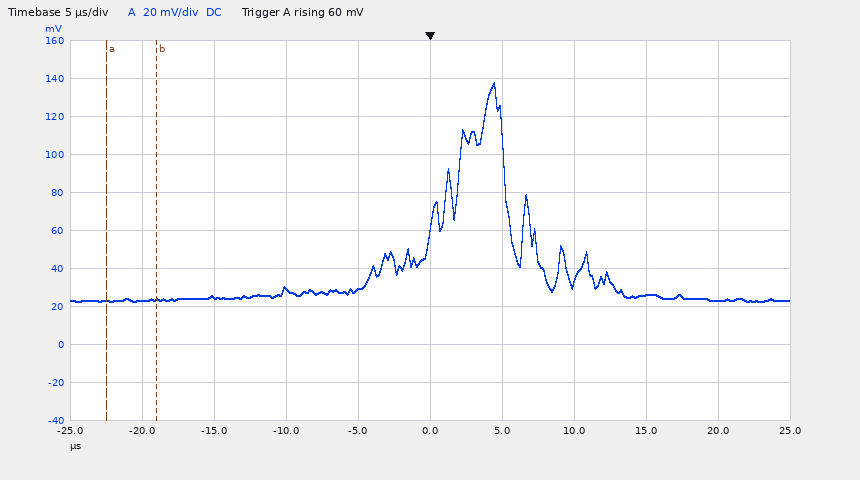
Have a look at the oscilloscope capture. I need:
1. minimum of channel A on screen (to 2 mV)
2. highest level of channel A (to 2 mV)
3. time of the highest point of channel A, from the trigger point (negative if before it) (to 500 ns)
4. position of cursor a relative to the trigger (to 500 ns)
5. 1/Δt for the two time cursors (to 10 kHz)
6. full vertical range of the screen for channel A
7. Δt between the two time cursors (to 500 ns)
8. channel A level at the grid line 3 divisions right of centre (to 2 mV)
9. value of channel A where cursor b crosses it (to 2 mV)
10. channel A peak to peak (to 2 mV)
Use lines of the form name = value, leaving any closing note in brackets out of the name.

minimum of channel A on screen = 22 mV
highest level of channel A = 138 mV
time of the highest point of channel A, from the trigger point (negative if before it) = +4.5 µs
position of cursor a relative to the trigger = -22.5 µs
1/Δt for the two time cursors = 290 kHz
full vertical range of the screen for channel A = 200 mV
Δt between the two time cursors = 3.5 µs
channel A level at the grid line 3 divisions right of centre = 26 mV
value of channel A where cursor b crosses it = 24 mV
channel A peak to peak = 116 mV
